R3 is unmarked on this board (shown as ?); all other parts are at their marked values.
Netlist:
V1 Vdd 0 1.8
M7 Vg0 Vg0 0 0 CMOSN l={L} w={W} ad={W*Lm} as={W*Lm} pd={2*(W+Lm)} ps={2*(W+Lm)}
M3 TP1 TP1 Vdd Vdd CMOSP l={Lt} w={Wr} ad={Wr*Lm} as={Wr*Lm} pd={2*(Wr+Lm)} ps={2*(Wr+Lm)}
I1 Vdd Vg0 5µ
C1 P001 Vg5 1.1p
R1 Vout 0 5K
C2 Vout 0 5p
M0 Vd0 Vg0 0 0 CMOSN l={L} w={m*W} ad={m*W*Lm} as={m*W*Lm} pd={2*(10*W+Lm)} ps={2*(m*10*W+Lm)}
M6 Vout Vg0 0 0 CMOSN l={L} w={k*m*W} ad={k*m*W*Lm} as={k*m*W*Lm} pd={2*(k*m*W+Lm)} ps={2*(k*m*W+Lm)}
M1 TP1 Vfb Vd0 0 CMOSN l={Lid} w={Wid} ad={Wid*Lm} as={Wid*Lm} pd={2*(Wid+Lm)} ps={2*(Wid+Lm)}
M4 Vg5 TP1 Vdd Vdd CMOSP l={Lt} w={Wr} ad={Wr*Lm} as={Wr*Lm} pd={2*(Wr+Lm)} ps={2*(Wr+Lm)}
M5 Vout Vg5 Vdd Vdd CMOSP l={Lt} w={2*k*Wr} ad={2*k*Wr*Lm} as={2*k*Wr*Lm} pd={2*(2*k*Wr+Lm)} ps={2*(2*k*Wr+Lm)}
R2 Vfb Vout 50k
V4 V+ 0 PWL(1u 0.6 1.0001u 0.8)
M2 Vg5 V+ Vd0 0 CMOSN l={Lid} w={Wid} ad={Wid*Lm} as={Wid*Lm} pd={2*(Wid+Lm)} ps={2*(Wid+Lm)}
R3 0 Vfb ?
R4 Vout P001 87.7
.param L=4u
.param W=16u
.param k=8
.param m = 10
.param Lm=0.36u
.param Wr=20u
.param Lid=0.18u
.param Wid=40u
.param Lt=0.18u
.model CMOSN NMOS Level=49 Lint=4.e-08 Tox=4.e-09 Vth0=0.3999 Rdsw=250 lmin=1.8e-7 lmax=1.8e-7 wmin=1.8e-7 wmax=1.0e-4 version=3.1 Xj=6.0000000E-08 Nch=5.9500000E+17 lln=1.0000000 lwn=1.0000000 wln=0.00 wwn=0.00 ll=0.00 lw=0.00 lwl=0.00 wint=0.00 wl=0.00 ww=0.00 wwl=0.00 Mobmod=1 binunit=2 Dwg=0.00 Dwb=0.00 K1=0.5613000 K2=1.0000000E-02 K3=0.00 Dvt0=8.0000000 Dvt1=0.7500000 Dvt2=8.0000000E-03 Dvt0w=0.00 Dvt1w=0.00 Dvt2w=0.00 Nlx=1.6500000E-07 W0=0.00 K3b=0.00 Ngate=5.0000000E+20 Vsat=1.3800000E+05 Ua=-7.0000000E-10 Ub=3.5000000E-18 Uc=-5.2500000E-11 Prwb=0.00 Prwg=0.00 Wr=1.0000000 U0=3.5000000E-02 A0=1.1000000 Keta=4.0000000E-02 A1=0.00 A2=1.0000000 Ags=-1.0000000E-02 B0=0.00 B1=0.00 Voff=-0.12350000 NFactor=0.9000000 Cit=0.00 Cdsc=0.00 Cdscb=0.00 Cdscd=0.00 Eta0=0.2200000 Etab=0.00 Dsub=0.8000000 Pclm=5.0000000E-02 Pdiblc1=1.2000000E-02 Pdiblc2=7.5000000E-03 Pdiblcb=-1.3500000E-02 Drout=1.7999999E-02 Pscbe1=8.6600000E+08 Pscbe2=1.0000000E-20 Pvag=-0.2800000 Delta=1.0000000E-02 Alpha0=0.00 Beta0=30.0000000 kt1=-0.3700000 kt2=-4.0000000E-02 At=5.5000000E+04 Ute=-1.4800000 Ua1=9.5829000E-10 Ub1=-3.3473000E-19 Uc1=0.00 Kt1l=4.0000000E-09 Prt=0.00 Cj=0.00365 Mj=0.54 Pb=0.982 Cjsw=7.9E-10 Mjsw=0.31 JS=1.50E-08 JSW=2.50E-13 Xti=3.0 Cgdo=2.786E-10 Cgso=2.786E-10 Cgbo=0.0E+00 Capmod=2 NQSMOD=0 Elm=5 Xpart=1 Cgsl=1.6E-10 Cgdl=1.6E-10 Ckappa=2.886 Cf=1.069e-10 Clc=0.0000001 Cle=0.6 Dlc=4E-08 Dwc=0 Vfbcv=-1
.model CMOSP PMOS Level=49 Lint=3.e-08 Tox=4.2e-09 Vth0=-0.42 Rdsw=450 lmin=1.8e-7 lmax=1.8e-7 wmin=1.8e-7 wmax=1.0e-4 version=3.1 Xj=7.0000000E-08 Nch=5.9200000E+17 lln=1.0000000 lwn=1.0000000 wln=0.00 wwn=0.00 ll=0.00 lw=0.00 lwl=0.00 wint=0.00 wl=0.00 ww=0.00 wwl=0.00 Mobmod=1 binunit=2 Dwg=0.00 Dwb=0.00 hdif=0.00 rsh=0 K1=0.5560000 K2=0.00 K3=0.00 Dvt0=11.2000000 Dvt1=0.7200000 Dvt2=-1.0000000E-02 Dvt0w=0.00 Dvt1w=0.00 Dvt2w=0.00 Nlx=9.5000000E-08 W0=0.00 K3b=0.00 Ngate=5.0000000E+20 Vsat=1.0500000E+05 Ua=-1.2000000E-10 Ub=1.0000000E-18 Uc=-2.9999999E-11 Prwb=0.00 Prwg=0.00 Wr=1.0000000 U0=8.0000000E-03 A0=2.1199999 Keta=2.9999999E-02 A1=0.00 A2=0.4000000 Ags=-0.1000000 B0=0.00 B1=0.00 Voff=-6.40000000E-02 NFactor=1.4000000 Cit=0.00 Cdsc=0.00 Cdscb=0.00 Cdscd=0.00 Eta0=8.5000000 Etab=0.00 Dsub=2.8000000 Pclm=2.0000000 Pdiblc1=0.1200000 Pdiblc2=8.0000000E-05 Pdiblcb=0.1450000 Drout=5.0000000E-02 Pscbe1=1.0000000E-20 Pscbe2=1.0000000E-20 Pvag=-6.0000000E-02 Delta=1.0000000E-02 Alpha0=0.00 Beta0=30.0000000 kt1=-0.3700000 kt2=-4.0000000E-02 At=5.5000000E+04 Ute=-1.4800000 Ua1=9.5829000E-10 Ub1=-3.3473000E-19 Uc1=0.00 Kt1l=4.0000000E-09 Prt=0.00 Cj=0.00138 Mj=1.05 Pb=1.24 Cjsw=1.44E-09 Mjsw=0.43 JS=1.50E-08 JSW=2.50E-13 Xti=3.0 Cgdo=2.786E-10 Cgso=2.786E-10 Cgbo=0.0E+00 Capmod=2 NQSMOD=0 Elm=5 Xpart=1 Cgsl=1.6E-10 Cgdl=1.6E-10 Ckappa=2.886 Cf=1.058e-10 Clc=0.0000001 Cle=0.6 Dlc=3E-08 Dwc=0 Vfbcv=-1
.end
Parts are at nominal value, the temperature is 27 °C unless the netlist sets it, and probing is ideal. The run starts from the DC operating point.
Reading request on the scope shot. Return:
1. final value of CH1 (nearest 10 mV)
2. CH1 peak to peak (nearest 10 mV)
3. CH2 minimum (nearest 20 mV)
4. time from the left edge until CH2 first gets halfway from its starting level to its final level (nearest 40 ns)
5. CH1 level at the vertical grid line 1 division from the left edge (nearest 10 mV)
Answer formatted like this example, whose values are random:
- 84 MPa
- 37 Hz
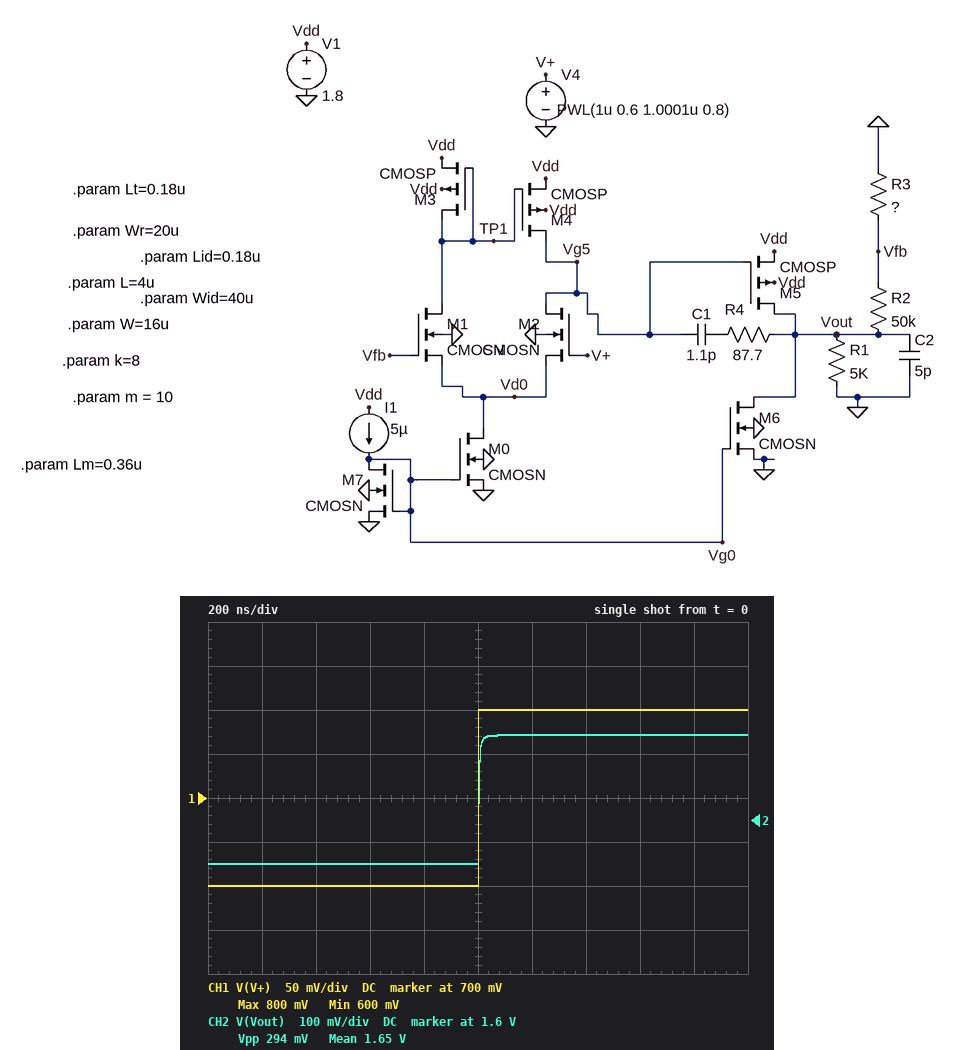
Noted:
- 800 mV
- 200 mV
- 1.50 V
- 1.00 µs
- 600 mV
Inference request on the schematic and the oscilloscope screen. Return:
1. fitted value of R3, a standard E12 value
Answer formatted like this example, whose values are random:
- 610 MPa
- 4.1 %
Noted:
- 33 kΩ
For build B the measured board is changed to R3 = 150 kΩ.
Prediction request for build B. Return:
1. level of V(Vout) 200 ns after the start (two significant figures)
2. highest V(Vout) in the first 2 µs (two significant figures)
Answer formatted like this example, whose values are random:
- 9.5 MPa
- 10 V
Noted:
- 800 mV
- 1.1 V
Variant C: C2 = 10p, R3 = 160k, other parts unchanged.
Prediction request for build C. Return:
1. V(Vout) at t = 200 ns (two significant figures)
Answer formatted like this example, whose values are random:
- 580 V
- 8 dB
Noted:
- 790 mV
